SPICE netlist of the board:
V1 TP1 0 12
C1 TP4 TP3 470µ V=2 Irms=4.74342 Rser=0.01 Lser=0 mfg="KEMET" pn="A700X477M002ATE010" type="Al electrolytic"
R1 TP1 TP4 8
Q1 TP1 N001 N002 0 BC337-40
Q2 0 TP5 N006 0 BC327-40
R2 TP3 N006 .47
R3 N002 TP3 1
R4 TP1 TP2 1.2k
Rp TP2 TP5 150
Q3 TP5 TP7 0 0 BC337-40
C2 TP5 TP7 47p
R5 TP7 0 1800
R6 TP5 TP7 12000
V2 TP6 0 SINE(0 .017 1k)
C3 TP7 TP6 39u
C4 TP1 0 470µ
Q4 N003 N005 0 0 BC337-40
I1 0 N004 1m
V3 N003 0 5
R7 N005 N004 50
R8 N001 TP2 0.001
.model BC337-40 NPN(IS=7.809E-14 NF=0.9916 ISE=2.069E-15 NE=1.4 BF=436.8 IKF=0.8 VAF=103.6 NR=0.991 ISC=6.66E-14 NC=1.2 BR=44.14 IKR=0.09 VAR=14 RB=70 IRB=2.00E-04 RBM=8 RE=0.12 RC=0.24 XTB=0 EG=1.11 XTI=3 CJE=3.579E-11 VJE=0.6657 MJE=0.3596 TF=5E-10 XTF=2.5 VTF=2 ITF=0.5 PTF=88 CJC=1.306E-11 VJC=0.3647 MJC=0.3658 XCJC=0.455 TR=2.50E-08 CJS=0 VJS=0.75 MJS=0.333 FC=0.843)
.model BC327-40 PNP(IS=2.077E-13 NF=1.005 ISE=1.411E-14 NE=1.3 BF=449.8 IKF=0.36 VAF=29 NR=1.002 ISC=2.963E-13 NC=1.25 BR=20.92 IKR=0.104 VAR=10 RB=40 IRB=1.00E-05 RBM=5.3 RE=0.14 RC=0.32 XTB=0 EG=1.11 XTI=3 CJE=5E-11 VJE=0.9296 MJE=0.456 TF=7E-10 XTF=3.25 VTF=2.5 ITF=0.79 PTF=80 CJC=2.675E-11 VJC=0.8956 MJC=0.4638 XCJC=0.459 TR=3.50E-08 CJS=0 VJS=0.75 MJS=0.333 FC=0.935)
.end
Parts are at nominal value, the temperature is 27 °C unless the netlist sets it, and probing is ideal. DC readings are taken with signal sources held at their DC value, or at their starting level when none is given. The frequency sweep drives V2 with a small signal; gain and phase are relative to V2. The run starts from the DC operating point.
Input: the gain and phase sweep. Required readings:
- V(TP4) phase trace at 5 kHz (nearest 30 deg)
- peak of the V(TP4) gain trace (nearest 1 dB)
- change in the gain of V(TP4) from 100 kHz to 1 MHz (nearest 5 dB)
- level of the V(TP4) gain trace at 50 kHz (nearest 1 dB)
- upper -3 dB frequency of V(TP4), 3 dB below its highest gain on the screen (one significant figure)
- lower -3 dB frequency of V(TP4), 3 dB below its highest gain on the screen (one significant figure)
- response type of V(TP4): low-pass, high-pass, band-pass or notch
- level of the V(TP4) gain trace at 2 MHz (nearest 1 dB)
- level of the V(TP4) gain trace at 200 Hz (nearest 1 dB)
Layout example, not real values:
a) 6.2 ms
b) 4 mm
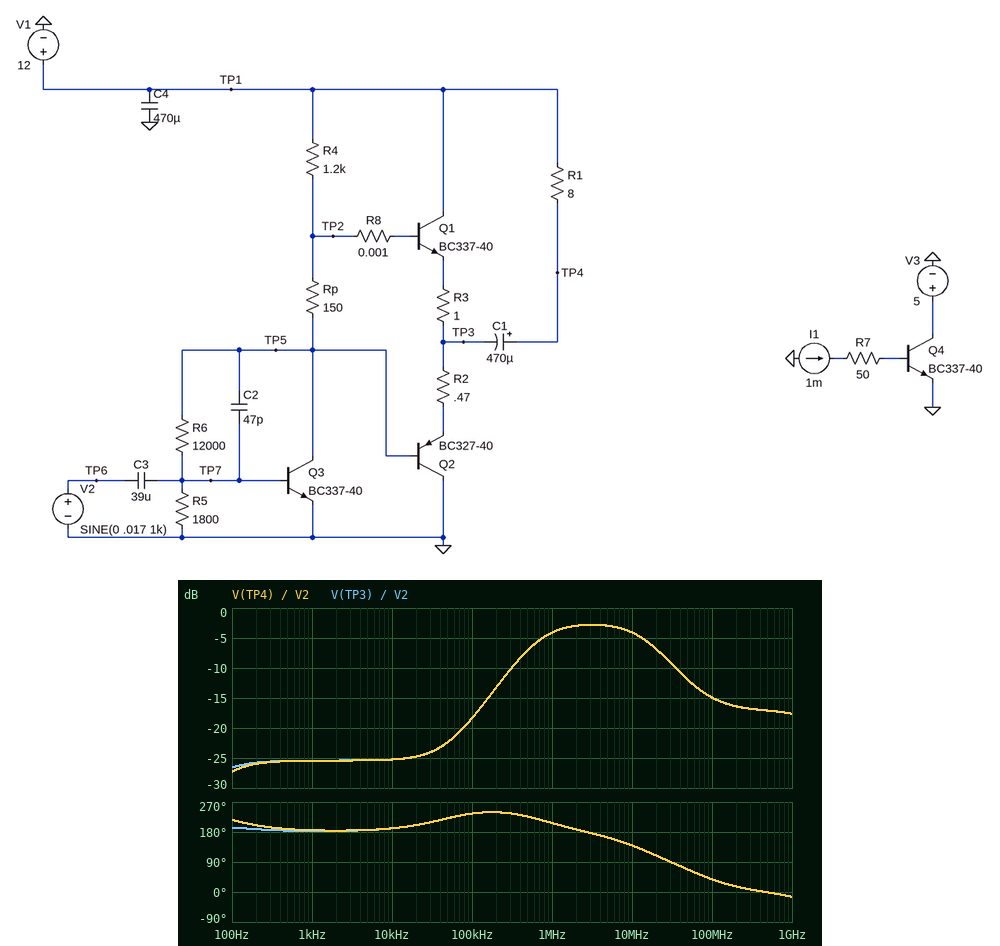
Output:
a) 180 deg
b) -3 dB
c) 15 dB
d) -22 dB
e) 20 MHz
f) 600 kHz
g) band-pass
h) -3 dB
i) -26 dB
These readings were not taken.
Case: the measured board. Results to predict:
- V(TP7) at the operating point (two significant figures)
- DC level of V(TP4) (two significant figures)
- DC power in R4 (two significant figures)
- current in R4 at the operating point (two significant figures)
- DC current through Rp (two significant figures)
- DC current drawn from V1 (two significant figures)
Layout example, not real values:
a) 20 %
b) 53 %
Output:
a) 640 mV
b) 12 V
c) 32 mW
d) 5.2 mA
e) 5.2 mA
f) 5.2 mA
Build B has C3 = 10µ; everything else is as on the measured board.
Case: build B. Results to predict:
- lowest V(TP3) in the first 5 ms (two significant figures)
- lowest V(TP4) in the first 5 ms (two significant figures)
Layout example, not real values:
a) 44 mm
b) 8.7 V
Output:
a) 3.2 V
b) 9.9 V
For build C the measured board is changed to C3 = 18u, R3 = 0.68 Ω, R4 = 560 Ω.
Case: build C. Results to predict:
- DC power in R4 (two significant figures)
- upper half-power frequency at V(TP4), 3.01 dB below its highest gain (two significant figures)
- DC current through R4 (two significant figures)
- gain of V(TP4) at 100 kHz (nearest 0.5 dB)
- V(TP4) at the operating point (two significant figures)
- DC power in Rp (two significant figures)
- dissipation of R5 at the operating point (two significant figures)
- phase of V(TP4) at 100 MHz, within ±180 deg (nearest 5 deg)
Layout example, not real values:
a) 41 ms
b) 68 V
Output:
a) 50 mW
b) 1.4 MHz
c) 9.5 mA
d) 43.0 dB
e) 12 V
f) 13 mW
g) 240 µW
h) -30 deg
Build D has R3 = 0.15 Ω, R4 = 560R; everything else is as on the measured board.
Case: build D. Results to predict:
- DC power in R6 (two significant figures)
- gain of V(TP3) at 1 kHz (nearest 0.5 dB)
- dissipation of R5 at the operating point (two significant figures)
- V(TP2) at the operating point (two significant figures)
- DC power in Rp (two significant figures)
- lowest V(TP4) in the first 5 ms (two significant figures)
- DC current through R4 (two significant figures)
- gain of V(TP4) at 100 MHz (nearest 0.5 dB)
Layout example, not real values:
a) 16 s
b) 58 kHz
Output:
a) 1.8 mW
b) 43.0 dB
c) 240 µW
d) 6.7 V
e) 13 mW
f) 9.8 V
g) 9.5 mA
h) -6.0 dB
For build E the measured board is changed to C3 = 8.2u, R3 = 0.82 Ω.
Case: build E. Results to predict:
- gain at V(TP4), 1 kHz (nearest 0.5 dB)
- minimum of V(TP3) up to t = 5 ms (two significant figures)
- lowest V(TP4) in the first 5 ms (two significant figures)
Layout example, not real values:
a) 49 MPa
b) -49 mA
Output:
a) -26.0 dB
b) 3.2 V
c) 9.9 V
